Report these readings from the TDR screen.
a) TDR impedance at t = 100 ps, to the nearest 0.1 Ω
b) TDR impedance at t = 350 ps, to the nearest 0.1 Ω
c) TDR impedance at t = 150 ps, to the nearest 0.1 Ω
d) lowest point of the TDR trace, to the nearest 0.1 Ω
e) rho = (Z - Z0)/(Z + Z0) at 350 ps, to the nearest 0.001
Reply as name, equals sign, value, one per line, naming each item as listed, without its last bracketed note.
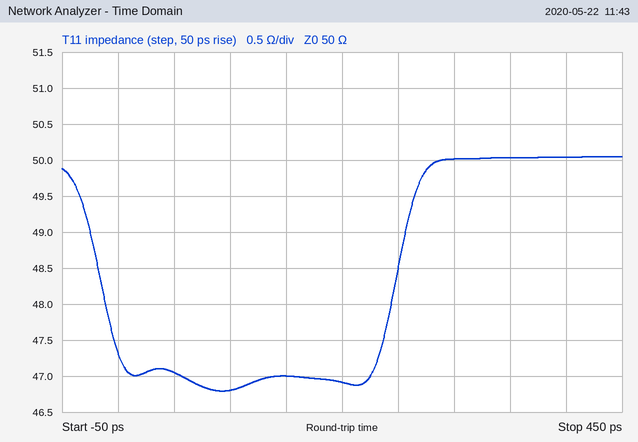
TDR impedance at t = 100 ps, to the nearest 0.1 Ω = 46.8 Ω
TDR impedance at t = 350 ps, to the nearest 0.1 Ω = 50.0 Ω
TDR impedance at t = 150 ps, to the nearest 0.1 Ω = 47.0 Ω
lowest point of the TDR trace, to the nearest 0.1 Ω = 46.8 Ω
rho = (Z - Z0)/(Z + Z0) at 350 ps, to the nearest 0.001 = 0.000
